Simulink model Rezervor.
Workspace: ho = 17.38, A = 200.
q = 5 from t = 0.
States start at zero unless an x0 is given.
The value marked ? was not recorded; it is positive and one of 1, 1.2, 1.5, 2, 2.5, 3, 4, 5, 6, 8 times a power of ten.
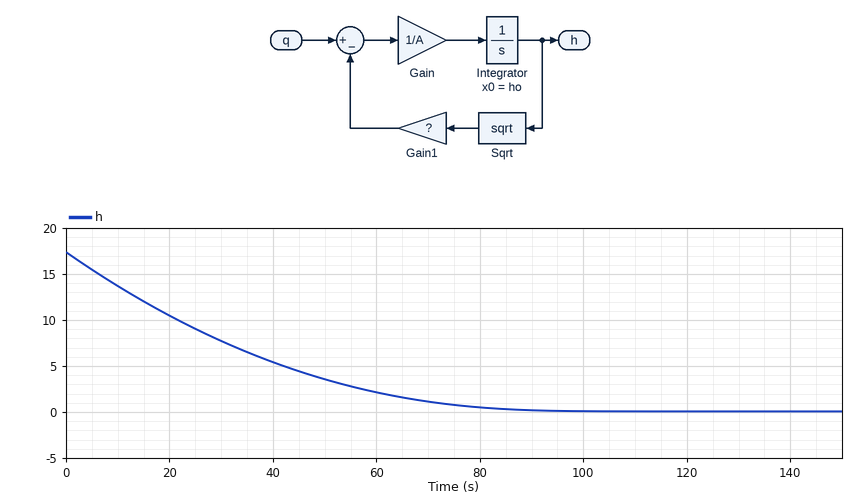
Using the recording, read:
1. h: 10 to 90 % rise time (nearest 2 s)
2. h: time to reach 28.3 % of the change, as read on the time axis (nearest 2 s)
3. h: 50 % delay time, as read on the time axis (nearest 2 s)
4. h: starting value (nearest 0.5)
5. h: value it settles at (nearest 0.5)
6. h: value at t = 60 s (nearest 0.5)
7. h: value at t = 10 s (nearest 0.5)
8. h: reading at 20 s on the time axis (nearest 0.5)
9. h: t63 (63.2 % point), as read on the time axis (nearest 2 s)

58 s
14 s
26 s
17.5
0.0
2.0
13.5
10.5
36 s
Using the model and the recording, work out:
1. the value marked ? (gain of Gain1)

20
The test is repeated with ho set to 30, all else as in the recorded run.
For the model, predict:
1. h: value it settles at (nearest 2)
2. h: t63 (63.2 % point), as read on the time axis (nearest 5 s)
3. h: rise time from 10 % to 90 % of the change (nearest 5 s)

0
45 s
75 s
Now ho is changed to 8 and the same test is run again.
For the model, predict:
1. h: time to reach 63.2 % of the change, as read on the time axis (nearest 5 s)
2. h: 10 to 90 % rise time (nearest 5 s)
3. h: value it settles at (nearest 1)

25 s
40 s
0
